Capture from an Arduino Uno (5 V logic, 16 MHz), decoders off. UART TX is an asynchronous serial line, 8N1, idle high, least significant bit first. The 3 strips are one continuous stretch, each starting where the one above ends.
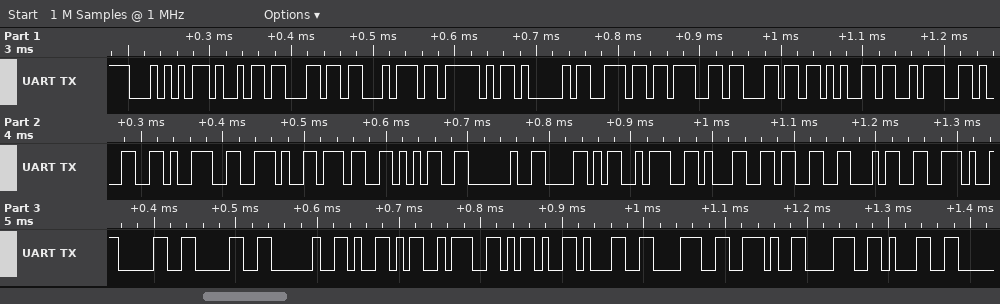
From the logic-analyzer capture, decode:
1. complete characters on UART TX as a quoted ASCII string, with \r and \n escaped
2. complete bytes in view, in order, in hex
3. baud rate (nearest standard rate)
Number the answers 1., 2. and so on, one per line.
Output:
1. "Tilt_Angle:19.75 X:134.00 Y:-18.81"
2. 0x54 0x69 0x6C 0x74 0x5F 0x41 0x6E 0x67 0x6C 0x65 0x3A 0x31 0x39 0x2E 0x37 0x35 0x20 0x58 0x3A 0x31 0x33 0x34 0x2E 0x30 0x30 0x20 0x59 0x3A 0x2D 0x31 0x38 0x2E 0x38 0x31
3. 115200 baud
